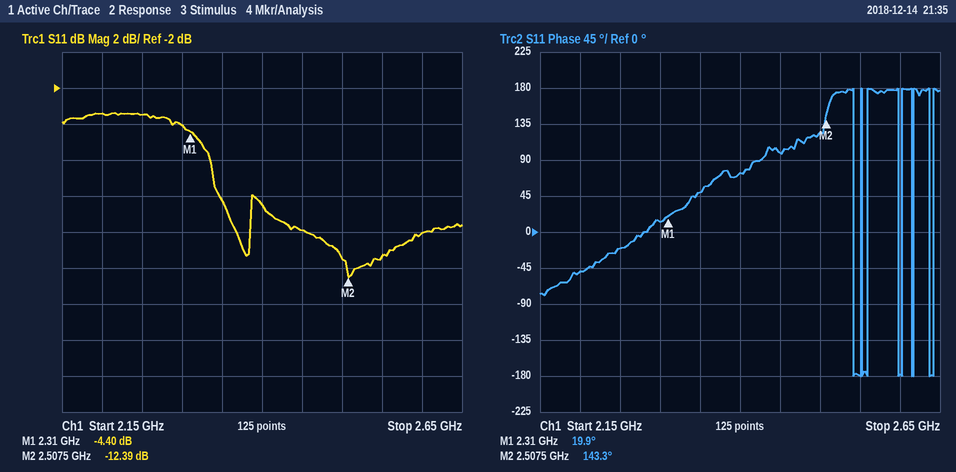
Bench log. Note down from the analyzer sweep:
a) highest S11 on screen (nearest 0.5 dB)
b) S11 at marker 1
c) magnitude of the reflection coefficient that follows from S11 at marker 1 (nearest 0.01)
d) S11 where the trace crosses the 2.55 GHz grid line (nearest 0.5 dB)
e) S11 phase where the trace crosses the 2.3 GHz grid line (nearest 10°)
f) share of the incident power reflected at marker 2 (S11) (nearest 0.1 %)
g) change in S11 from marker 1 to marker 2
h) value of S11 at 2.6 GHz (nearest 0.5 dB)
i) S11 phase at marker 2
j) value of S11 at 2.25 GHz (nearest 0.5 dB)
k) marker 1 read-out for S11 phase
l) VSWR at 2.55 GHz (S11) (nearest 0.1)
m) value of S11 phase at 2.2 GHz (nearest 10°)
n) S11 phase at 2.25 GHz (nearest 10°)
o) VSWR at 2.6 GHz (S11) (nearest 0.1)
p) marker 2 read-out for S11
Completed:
-3.5 dB
-4.40 dB
0.60
-11.5 dB
10°
5.8 %
-7.99 dB
-10.0 dB
143.3°
-3.5 dB
19.9°
1.7
-50°
-20°
1.9
-12.39 dB
